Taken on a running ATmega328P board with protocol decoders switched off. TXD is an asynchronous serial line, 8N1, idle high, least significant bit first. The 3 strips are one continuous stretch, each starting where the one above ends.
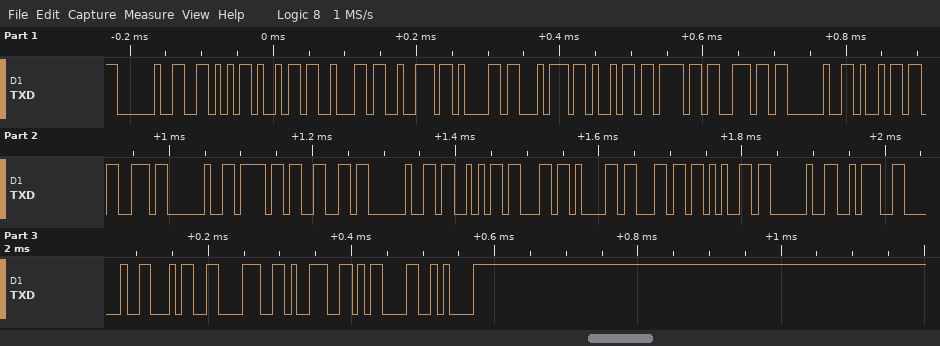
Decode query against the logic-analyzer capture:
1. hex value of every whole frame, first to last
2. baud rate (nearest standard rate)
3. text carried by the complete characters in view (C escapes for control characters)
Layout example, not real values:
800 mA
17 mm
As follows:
20 56 69 62 72 61 74 69 6F 6E 20 69 73 20 6F 66 20 53 63 61 6C 65 20 3A 20 34 38 39 0D 0A
115200 baud
" Vibration is of Scale : 489\r\n"
